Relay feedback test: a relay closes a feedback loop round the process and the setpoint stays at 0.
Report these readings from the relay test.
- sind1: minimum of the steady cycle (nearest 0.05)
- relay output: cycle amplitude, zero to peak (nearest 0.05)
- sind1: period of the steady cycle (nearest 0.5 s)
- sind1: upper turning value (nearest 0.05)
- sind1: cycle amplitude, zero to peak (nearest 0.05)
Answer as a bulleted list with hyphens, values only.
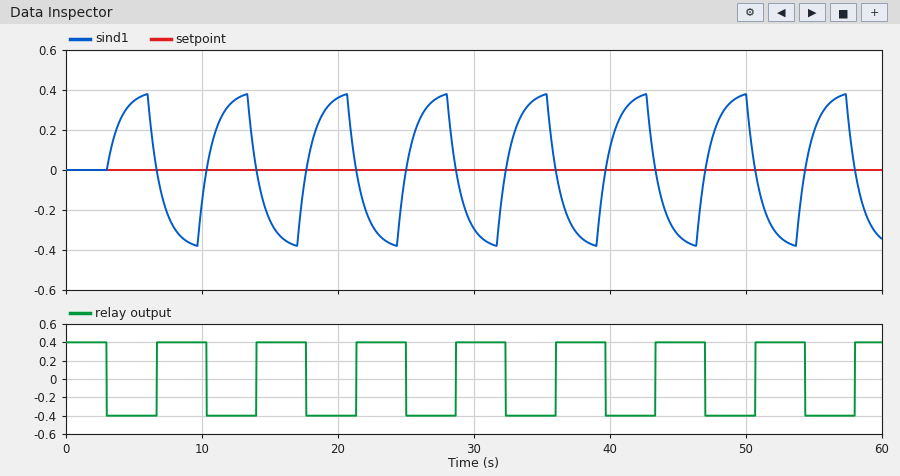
- -0.40
- 0.40
- 7.5 s
- 0.40
- 0.40
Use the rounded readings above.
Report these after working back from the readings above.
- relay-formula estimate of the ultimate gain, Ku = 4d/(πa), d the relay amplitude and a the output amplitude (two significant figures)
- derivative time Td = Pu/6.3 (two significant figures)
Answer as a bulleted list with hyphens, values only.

- 1.3
- 1.2 s
